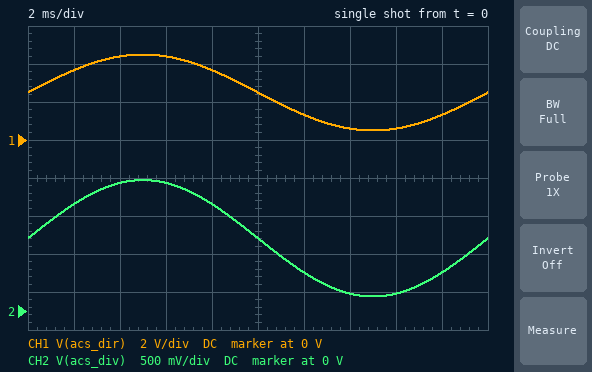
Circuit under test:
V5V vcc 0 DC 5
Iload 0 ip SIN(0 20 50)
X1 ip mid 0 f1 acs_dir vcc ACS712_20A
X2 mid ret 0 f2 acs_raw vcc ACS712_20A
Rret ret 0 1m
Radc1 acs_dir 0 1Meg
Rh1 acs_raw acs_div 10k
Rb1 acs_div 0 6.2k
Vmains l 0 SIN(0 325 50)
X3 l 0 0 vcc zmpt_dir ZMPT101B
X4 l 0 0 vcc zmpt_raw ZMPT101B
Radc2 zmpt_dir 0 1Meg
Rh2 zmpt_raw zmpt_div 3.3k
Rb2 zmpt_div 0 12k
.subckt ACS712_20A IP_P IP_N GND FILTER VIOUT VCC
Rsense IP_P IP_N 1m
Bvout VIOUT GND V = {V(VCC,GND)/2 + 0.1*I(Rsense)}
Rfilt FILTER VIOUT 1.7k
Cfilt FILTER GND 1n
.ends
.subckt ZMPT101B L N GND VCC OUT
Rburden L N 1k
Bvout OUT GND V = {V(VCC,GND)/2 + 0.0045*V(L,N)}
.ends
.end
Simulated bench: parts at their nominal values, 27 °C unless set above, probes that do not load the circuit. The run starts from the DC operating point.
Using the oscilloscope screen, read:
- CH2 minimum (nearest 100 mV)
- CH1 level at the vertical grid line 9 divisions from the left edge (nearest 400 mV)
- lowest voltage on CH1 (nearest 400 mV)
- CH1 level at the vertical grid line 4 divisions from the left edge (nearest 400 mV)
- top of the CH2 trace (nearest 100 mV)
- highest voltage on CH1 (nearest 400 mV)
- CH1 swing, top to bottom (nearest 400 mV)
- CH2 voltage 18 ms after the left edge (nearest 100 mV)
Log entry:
200 mV
1.2 V
400 mV
3.6 V
1.7 V
4.4 V
4.0 V
500 mV
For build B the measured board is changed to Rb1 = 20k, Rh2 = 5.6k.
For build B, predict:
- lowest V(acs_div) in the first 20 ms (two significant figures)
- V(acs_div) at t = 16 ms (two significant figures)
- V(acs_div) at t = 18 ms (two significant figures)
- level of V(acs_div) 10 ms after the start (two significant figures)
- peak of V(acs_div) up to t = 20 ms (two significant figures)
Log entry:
330 mV
400 mV
880 mV
1.7 V
3.0 V
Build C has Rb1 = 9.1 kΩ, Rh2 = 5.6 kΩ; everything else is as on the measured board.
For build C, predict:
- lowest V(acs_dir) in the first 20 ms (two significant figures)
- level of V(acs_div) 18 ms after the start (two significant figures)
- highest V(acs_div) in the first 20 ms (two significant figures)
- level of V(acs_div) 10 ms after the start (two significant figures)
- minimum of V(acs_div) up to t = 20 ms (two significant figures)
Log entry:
500 mV
630 mV
2.1 V
1.2 V
240 mV
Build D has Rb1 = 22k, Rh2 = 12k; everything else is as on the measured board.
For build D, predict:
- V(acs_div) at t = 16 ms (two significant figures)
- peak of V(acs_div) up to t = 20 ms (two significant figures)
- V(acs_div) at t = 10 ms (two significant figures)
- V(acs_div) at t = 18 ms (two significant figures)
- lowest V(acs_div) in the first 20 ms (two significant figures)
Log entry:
410 mV
3.1 V
1.7 V
910 mV
340 mV
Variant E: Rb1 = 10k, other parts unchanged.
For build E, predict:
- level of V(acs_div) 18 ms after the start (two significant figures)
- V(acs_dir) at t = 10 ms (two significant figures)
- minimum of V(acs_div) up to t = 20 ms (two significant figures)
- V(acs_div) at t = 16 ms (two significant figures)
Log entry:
660 mV
2.5 V
250 mV
300 mV
